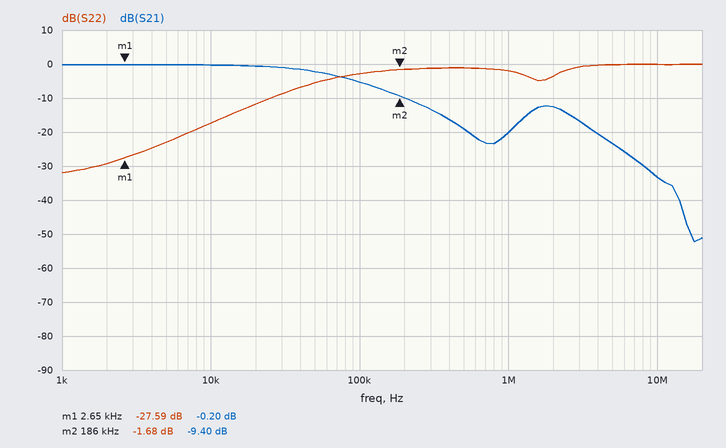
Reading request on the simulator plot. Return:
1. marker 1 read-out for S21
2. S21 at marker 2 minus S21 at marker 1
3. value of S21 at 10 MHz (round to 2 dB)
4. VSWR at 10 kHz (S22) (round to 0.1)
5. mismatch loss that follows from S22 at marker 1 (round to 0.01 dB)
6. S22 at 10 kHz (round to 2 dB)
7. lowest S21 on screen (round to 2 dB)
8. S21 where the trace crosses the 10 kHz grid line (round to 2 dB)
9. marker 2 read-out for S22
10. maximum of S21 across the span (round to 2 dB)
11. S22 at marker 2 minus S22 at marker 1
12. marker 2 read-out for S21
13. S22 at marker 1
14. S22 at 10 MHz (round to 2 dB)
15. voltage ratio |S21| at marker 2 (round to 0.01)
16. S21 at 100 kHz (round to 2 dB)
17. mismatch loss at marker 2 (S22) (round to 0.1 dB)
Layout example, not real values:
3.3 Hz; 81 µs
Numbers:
-0.20 dB; -9.20 dB; -34 dB; 1.3; 0.01 dB; -18 dB; -52 dB; 0 dB; -1.68 dB; 0 dB; 25.91 dB; -9.40 dB; -27.59 dB; 0 dB; 0.34; -6 dB; 4.9 dB
